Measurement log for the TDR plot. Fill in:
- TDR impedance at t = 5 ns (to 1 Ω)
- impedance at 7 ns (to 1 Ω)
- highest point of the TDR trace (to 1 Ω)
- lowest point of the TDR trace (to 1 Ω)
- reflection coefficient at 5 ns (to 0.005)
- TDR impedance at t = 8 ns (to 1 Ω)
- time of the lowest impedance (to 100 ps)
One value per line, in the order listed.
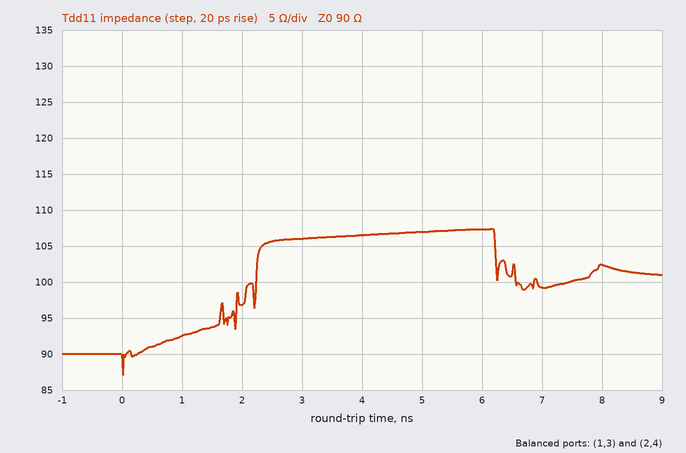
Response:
107 Ω
99 Ω
107 Ω
87 Ω
+0.085
102 Ω
0.0 ns
